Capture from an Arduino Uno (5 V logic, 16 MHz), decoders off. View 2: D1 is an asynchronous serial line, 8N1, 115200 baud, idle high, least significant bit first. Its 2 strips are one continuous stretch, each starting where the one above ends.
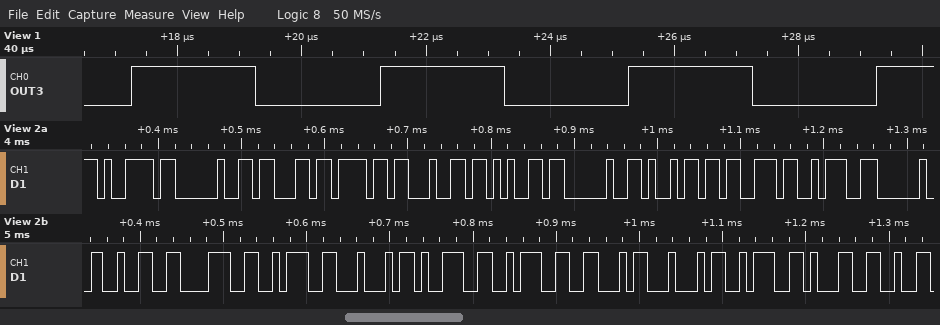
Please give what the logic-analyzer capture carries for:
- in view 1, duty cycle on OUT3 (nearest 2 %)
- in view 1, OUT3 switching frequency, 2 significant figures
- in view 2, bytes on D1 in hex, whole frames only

50 %
250 kHz
0x79 0x20 0x63 0x6F 0x64 0x65 0x20 0x69 0x73 0x3A 0x20 0x32 0x38 0x3A 0x44 0x39 0x3A 0x46 0x44 0x3A 0x31
